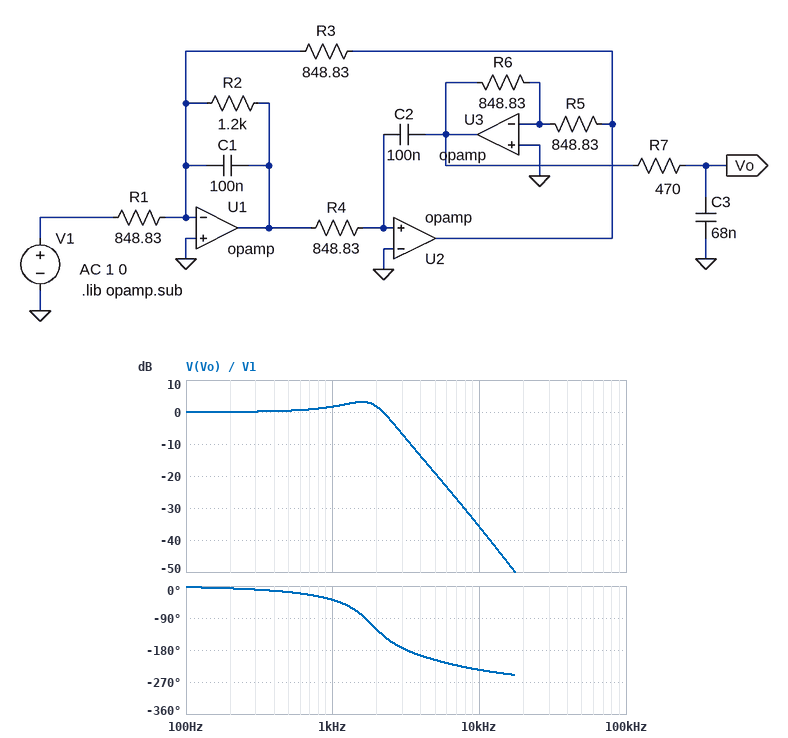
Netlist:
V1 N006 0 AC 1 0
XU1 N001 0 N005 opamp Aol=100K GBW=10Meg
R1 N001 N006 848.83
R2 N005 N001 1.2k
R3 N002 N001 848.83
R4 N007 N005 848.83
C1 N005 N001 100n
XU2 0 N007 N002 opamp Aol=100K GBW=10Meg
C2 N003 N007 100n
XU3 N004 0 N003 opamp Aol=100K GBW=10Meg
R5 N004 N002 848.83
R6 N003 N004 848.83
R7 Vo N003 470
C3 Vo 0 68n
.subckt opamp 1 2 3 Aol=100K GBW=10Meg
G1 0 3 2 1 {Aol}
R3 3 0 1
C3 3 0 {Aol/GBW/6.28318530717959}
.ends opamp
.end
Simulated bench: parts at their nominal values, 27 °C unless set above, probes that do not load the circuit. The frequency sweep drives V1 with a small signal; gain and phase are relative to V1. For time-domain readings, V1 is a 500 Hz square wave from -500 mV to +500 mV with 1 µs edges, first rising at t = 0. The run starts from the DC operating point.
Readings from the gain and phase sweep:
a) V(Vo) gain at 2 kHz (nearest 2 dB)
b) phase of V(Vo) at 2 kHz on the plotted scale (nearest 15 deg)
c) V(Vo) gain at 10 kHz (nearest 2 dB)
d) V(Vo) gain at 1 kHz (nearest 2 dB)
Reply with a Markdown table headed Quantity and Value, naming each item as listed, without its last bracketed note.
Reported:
| Quantity | Value |
|---|---|
| V(Vo) gain at 2 kHz | 2 dB |
| phase of V(Vo) at 2 kHz on the plotted scale | -120 deg |
| V(Vo) gain at 10 kHz | -36 dB |
| V(Vo) gain at 1 kHz | 2 dB |
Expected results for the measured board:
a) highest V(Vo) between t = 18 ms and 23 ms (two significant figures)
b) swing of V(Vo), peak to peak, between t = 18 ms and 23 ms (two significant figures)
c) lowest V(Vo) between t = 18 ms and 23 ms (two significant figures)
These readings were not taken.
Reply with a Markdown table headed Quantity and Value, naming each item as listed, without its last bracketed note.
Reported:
| Quantity | Value |
|---|---|
| highest V(Vo) between t = 18 ms and 23 ms | 780 mV |
| swing of V(Vo), peak to peak, between t = 18 ms and 23 ms | 1.6 V |
| lowest V(Vo) between t = 18 ms and 23 ms | -780 mV |
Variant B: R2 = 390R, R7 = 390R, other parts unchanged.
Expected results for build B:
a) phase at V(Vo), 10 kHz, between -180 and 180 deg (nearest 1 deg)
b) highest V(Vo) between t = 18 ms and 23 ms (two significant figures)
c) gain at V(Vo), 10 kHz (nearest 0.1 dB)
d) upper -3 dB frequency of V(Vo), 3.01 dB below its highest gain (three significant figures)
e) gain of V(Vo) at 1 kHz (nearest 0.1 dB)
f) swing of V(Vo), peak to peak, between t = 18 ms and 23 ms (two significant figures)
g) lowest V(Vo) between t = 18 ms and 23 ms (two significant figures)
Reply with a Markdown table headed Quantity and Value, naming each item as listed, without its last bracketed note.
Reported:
| Quantity | Value |
|---|---|
| phase at V(Vo), 10 kHz, between -180 and 180 deg | 144 deg |
| highest V(Vo) between t = 18 ms and 23 ms | 500 mV |
| gain at V(Vo), 10 kHz | -35.3 dB |
| upper -3 dB frequency of V(Vo), 3.01 dB below its highest gain | 1.04 kHz |
| gain of V(Vo) at 1 kHz | -2.8 dB |
| swing of V(Vo), peak to peak, between t = 18 ms and 23 ms | 1.0 V |
| lowest V(Vo) between t = 18 ms and 23 ms | -500 mV |
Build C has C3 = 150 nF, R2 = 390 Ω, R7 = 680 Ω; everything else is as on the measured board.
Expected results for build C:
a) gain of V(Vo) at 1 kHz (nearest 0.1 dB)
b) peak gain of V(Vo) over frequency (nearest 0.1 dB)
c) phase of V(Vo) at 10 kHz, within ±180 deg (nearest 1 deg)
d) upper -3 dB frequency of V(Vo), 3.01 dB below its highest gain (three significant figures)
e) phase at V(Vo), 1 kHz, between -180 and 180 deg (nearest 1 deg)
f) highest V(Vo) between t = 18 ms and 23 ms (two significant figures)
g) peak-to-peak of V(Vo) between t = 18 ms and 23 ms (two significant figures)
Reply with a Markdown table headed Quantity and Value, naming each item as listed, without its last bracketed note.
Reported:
| Quantity | Value |
|---|---|
| gain of V(Vo) at 1 kHz | -4.2 dB |
| peak gain of V(Vo) over frequency | 0 dB |
| phase of V(Vo) at 10 kHz, within ±180 deg | 122 deg |
| upper -3 dB frequency of V(Vo), 3.01 dB below its highest gain | 823 Hz |
| phase at V(Vo), 1 kHz, between -180 and 180 deg | -91 deg |
| highest V(Vo) between t = 18 ms and 23 ms | 500 mV |
| peak-to-peak of V(Vo) between t = 18 ms and 23 ms | 990 mV |
